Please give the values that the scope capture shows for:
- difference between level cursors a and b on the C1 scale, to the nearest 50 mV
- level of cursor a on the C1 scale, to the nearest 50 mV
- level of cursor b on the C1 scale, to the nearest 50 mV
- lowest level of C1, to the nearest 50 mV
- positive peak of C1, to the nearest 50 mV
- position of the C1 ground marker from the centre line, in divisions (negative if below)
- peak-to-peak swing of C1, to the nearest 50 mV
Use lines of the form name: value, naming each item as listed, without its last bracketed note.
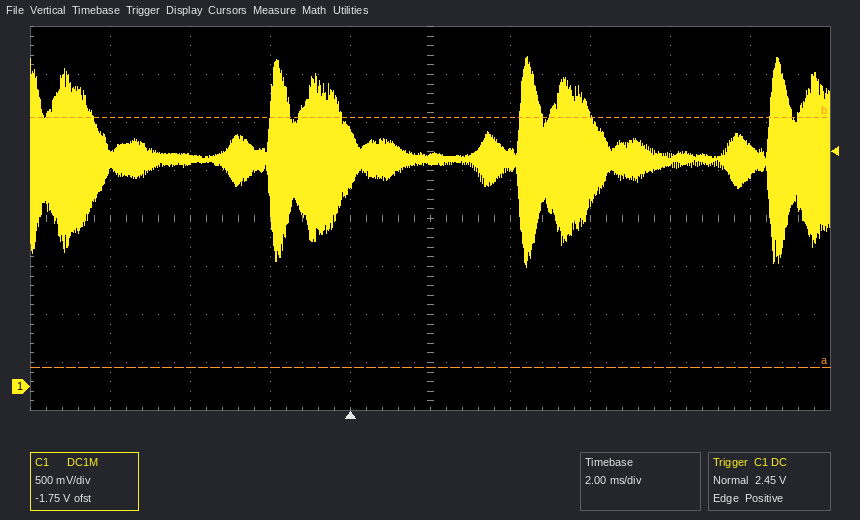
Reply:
difference between level cursors a and b on the C1 scale, to the nearest 50 mV: 2.60 V
level of cursor a on the C1 scale, to the nearest 50 mV: 200 mV
level of cursor b on the C1 scale, to the nearest 50 mV: 2.80 V
lowest level of C1, to the nearest 50 mV: 1.25 V
positive peak of C1, to the nearest 50 mV: 3.45 V
position of the C1 ground marker from the centre line, in divisions: -3.5 div
peak-to-peak swing of C1, to the nearest 50 mV: 2.20 V
